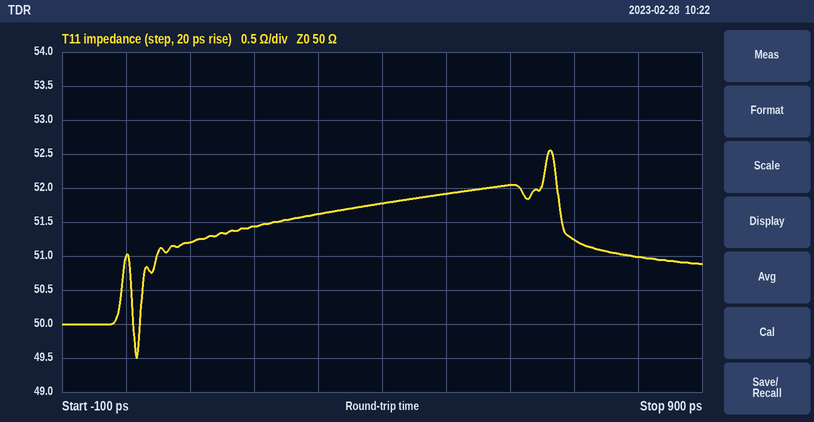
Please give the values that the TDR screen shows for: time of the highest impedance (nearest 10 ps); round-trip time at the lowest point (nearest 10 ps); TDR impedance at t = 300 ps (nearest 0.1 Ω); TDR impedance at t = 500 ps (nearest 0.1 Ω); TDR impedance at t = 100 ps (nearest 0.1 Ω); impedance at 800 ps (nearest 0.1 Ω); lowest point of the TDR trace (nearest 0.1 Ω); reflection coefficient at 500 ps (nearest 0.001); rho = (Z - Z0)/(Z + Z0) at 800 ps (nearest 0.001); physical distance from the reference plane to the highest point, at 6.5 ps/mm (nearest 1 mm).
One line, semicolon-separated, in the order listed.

660 ps; 20 ps; 51.6 Ω; 51.9 Ω; 51.2 Ω; 51.0 Ω; 49.5 Ω; +0.019; +0.010; 51 mm
